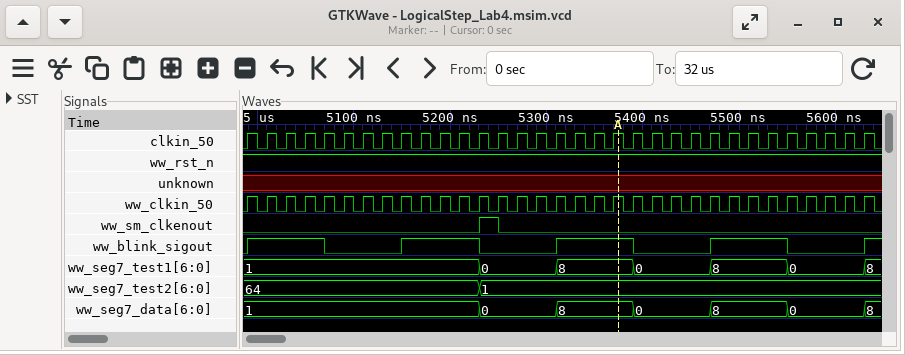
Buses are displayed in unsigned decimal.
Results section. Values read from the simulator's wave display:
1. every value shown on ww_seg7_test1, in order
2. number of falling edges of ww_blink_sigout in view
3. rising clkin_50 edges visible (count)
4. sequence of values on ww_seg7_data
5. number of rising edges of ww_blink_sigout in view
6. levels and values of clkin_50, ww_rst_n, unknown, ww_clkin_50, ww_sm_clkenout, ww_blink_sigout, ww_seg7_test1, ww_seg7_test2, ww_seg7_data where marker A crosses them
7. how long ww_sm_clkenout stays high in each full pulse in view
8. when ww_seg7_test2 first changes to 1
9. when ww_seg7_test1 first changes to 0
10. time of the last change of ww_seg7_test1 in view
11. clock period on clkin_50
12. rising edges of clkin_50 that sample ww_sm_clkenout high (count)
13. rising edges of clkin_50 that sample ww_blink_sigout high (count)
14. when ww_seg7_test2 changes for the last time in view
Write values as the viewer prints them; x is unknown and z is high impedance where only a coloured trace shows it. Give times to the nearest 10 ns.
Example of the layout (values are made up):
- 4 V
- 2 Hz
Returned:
- 1, 0, 8, 0, 8, 0, 8
- 4
- 33
- 1, 0, 8, 0, 8, 0, 8
- 5
- clkin_50=1, ww_rst_n=1, unknown=x, ww_clkin_50=1, ww_sm_clkenout=0, ww_blink_sigout=1, ww_seg7_test1=8, ww_seg7_test2=1, ww_seg7_data=8
- 20 ns
- 5230 ns
- 5230 ns
- 5630 ns
- 20 ns
- 1
- 16
- 5230 ns
